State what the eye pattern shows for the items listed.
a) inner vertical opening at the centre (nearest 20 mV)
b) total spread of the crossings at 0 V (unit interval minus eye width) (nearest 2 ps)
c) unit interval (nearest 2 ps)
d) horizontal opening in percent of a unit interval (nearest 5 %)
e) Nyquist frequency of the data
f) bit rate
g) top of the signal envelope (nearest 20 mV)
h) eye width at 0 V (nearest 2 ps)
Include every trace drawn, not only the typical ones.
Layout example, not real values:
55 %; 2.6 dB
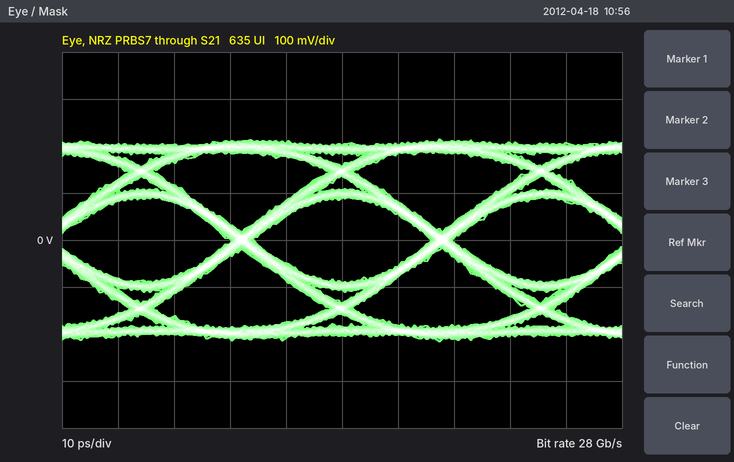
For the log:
180 mV; 4 ps; 36 ps; 90 %; 14 GHz; 28 Gb/s; 220 mV; 32 ps
